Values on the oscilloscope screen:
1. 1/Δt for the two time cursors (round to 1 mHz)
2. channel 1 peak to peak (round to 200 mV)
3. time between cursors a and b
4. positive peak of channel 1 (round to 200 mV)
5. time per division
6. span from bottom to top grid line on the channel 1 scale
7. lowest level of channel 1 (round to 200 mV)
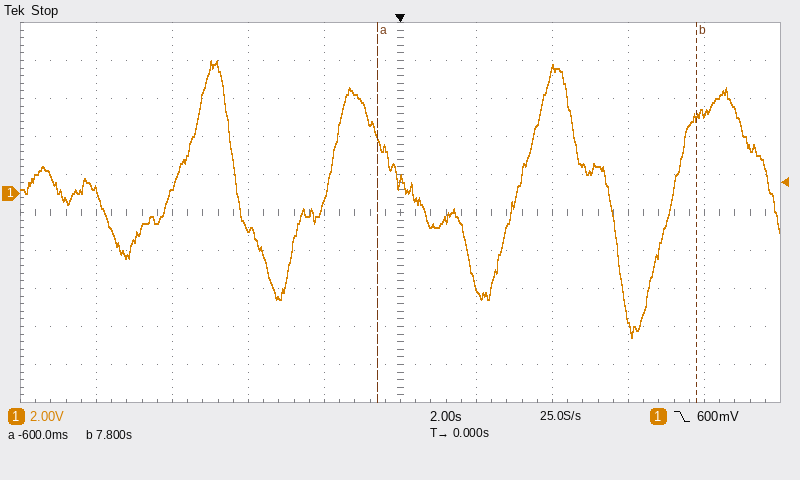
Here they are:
119 mHz
14.6 V
8.4 s
7.0 V
2 s
20 V
-7.6 V
